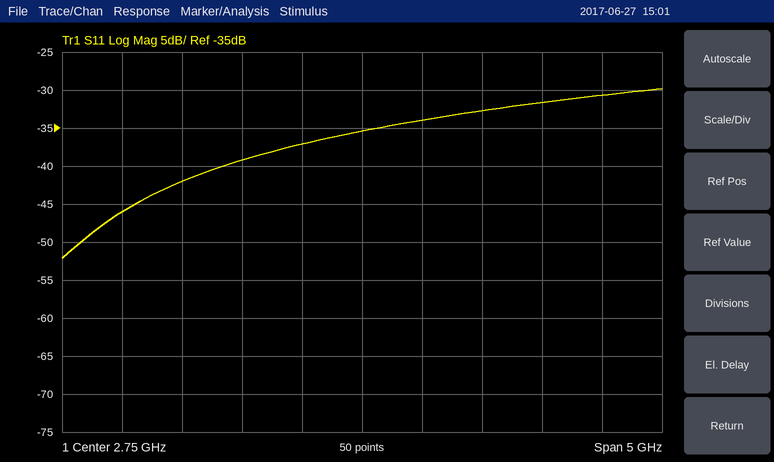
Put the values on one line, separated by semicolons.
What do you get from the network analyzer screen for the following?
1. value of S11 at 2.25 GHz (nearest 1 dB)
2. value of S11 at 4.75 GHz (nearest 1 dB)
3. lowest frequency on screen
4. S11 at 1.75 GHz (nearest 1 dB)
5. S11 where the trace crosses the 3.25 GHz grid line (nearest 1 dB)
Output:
-37 dB; -31 dB; 250 MHz; -39 dB; -34 dB
